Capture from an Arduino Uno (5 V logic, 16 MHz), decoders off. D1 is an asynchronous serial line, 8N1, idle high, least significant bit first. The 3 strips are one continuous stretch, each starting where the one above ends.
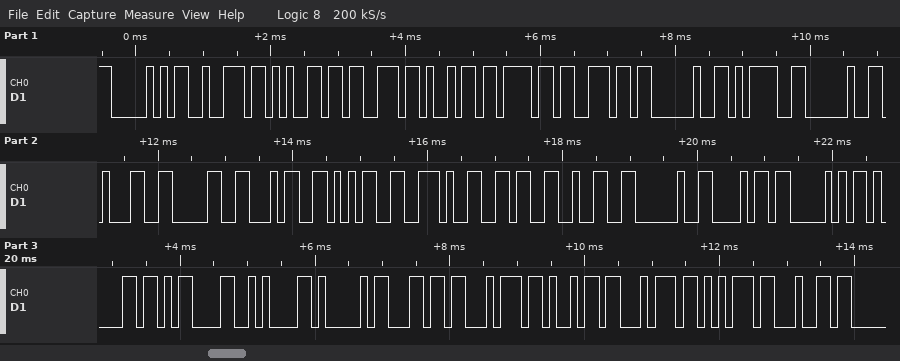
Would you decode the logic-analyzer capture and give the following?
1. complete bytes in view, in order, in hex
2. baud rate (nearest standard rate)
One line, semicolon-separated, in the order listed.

50 72 65 73 69 6F 6E 20 3D 20 31 30 34 35 2E 36 32 20 68 50 61 0D 0A 41 6C 74 69 74 75 64; 9600 baud
